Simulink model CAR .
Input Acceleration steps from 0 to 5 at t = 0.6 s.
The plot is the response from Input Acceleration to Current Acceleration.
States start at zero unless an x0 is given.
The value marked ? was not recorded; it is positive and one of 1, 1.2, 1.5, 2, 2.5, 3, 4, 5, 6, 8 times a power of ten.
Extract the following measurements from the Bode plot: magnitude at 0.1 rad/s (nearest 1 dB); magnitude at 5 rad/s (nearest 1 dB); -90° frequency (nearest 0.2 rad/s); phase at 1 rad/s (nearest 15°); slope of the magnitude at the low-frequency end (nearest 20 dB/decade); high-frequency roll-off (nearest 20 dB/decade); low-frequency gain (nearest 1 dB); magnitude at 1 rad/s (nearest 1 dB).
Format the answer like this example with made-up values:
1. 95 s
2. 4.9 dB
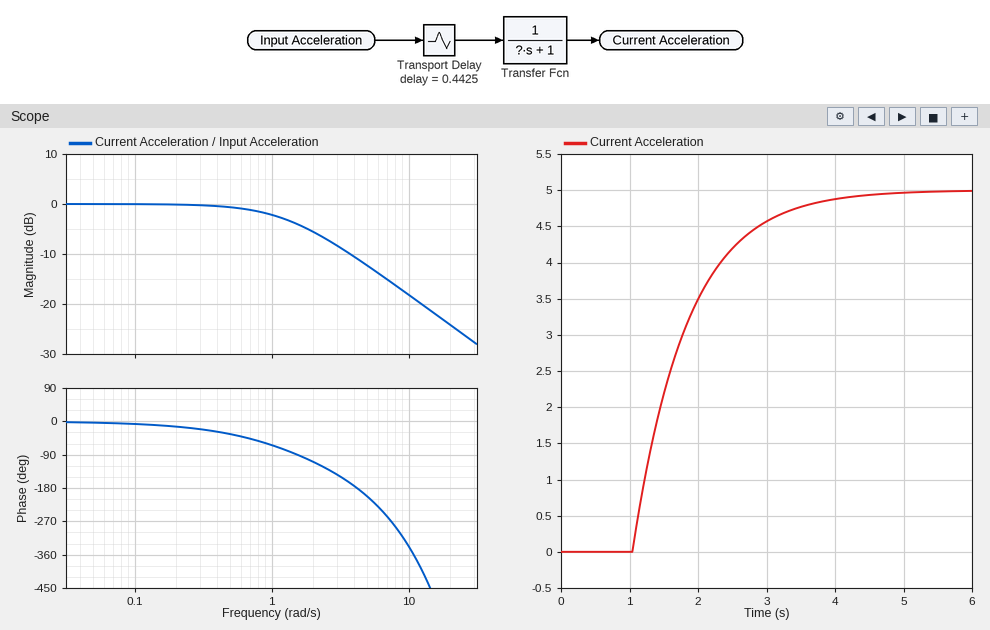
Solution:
1. 0 dB
2. -12 dB
3. 1.6 rad/s
4. -60°
5. 0 dB/decade
6. -20 dB/decade
7. 0 dB
8. -2 dB
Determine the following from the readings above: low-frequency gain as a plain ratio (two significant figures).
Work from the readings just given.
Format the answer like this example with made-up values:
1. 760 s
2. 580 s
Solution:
1. 1.0
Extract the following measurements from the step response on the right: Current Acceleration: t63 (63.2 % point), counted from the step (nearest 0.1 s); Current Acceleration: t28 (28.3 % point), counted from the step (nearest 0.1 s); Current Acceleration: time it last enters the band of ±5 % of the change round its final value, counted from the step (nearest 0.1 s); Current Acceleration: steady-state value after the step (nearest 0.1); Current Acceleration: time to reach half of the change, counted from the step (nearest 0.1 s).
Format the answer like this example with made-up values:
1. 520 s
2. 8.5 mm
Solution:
1. 1.2 s
2. 0.7 s
3. 2.8 s
4. 5.0
5. 1.0 s
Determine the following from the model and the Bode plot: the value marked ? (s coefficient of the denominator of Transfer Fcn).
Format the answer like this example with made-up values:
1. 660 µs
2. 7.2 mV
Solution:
1. 0.8
